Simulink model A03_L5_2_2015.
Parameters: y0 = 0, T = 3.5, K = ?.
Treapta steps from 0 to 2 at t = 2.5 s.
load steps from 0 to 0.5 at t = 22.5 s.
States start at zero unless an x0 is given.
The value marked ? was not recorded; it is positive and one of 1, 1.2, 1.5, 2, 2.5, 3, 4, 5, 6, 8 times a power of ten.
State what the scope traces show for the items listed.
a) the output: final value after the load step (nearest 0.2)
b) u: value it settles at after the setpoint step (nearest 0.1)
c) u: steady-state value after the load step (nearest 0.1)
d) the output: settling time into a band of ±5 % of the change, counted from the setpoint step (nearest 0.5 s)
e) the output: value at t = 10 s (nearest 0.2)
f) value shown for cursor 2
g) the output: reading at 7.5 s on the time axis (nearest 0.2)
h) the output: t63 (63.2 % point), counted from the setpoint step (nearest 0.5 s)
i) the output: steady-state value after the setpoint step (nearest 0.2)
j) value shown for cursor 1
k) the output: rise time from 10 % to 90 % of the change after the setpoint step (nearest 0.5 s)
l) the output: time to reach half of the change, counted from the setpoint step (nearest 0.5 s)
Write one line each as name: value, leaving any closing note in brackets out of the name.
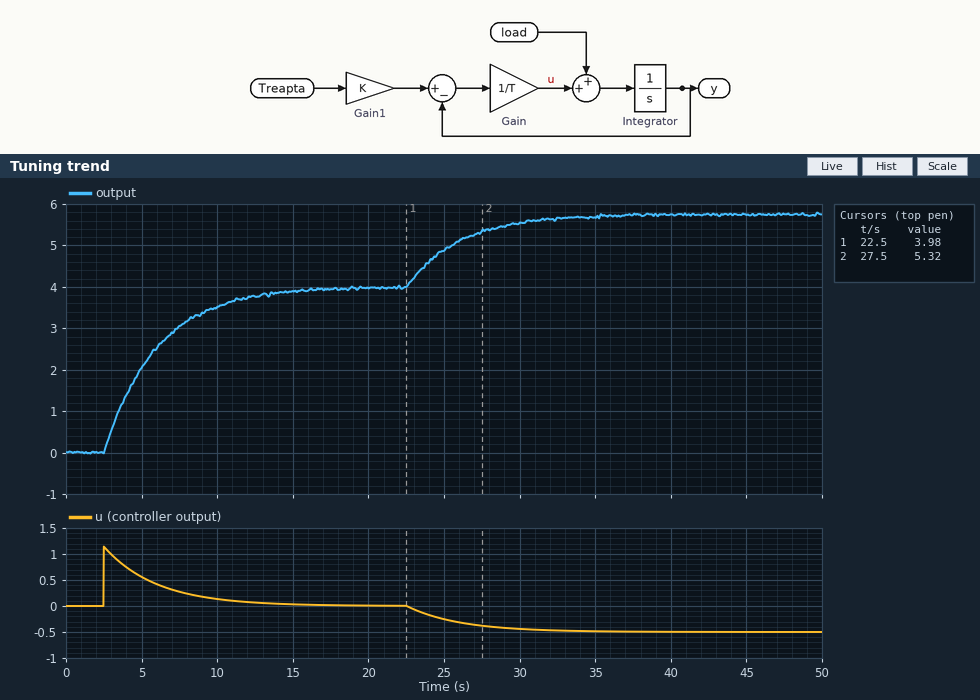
the output: final value after the load step: 5.8
u: value it settles at after the setpoint step: 0.0
u: steady-state value after the load step: -0.5
the output: settling time into a band of ±5 % of the change, counted from the setpoint step: 10.5 s
the output: value at t = 10 s: 3.6
value shown for cursor 2: 5.32
the output: reading at 7.5 s on the time axis: 3.0
the output: t63 (63.2 % point), counted from the setpoint step: 3.5 s
the output: steady-state value after the setpoint step: 4.0
value shown for cursor 1: 3.98
the output: rise time from 10 % to 90 % of the change after the setpoint step: 7.5 s
the output: time to reach half of the change, counted from the setpoint step: 2.5 s
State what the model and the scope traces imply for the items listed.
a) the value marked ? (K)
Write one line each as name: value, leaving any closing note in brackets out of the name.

the value marked ?: 2
